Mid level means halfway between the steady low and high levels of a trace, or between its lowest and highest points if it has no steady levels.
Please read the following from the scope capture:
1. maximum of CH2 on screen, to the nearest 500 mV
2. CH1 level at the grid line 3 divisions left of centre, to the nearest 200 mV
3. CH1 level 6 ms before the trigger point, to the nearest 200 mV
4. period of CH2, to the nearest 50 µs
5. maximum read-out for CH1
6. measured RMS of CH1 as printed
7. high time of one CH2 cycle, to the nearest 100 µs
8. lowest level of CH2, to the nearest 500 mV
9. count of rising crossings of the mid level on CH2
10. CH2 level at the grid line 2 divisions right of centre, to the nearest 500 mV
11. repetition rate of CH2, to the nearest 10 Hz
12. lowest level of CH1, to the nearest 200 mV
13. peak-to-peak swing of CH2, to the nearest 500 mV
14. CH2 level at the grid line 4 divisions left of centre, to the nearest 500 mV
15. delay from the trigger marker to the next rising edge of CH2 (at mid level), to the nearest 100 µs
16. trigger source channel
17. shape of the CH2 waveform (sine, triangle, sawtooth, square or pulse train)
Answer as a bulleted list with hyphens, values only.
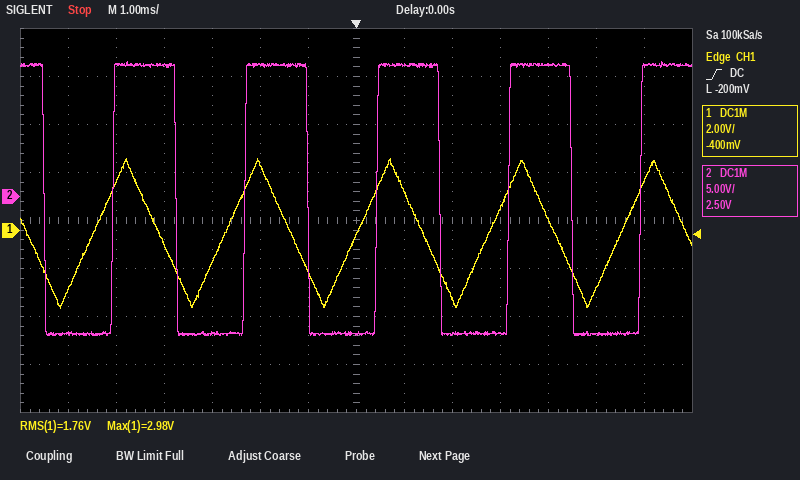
- 14.0 V
- -1.4 V
- -2.4 V
- 2.75 ms
- 2.98 V
- 1.76 V
- 1.3 ms
- -14.5 V
- 5
- -14.5 V
- 360 Hz
- -3.2 V
- 28.5 V
- 13.5 V
- 400 µs
- CH1
- square
